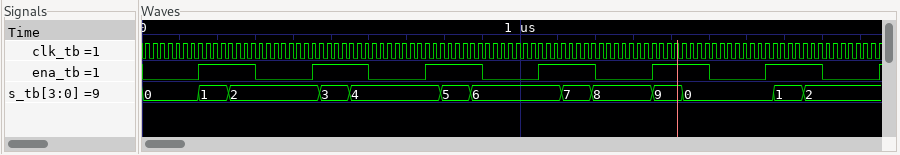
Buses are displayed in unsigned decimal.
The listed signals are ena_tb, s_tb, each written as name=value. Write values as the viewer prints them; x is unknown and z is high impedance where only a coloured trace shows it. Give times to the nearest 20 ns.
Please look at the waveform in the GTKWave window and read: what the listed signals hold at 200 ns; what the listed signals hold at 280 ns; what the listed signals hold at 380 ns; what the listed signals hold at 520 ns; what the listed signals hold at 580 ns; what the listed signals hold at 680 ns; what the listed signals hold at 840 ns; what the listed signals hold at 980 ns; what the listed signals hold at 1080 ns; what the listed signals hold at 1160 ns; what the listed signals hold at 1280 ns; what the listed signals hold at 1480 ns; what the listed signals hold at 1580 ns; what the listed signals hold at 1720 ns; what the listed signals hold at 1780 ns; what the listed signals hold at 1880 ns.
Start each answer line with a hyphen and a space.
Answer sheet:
- ena_tb=1, s_tb=1
- ena_tb=1, s_tb=2
- ena_tb=0, s_tb=2
- ena_tb=1, s_tb=3
- ena_tb=1, s_tb=4
- ena_tb=0, s_tb=4
- ena_tb=1, s_tb=5
- ena_tb=0, s_tb=6
- ena_tb=1, s_tb=6
- ena_tb=1, s_tb=7
- ena_tb=0, s_tb=8
- ena_tb=1, s_tb=0
- ena_tb=0, s_tb=0
- ena_tb=1, s_tb=1
- ena_tb=1, s_tb=2
- ena_tb=0, s_tb=2
